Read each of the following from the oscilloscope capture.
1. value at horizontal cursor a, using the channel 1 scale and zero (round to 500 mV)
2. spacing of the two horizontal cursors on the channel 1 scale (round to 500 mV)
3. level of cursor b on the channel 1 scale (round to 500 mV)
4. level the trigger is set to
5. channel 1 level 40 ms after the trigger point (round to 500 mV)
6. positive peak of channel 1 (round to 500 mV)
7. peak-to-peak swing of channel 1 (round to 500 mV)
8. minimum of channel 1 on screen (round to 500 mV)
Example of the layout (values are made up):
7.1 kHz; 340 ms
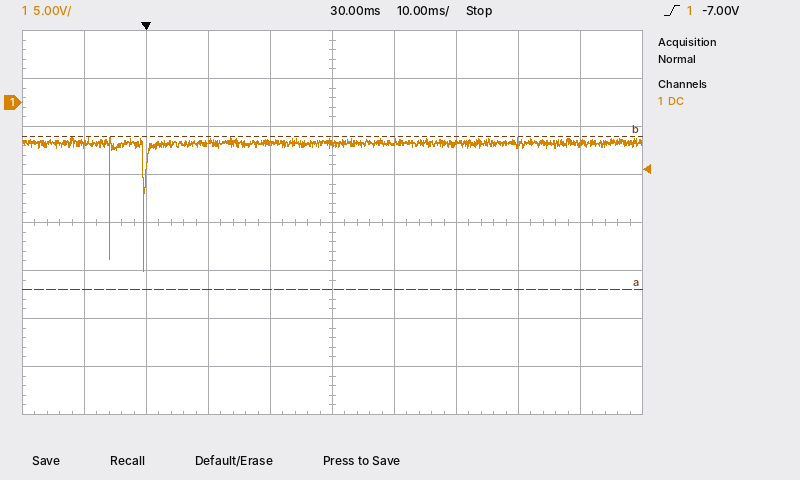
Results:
-19.5 V; 16.0 V; -3.5 V; -7.00 V; -4.0 V; -3.5 V; 14.0 V; -17.5 V
